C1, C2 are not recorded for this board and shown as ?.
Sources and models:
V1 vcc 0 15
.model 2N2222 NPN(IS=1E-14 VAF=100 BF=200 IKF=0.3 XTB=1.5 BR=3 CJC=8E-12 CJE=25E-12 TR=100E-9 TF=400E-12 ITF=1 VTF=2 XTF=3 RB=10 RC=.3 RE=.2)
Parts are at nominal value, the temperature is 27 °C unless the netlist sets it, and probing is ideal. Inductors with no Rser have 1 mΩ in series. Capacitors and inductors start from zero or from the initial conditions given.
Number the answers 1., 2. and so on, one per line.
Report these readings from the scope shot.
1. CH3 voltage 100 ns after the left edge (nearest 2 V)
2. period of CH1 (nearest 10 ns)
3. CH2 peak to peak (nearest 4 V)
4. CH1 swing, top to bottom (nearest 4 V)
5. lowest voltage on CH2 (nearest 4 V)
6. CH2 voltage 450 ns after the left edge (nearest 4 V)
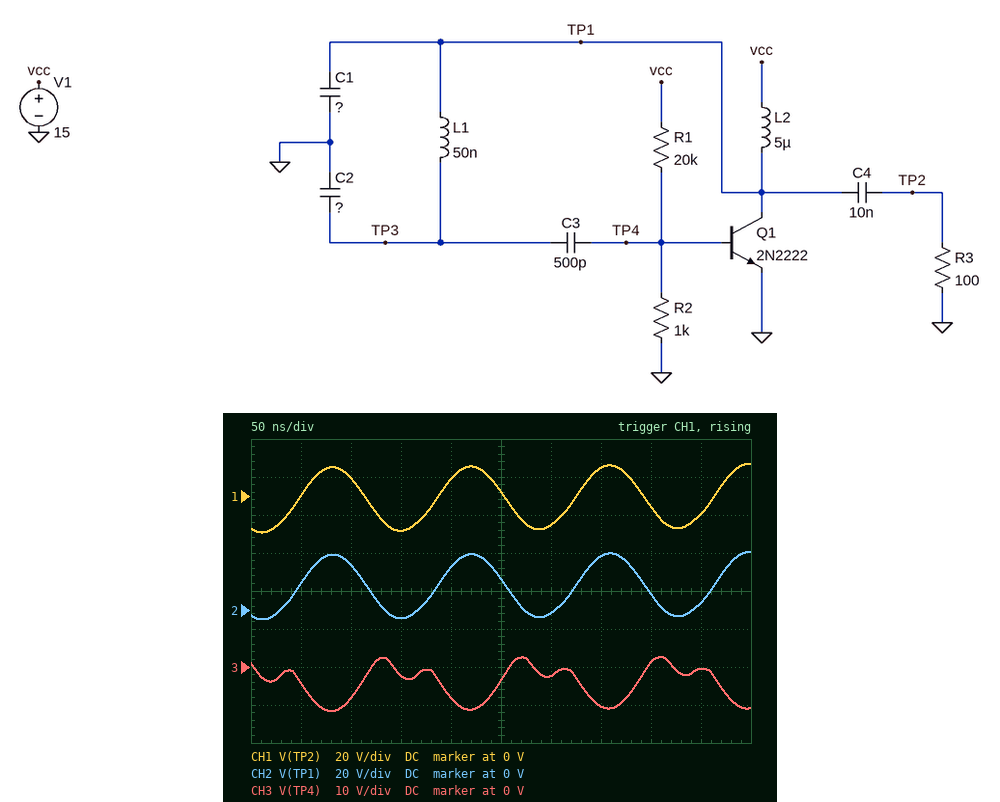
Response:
1. -8 V
2. 140 ns
3. 36 V
4. 36 V
5. -4 V
6. 4 V
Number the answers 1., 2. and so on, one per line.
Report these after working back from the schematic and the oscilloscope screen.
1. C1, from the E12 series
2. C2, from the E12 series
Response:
1. 15 nF
2. 27 nF
